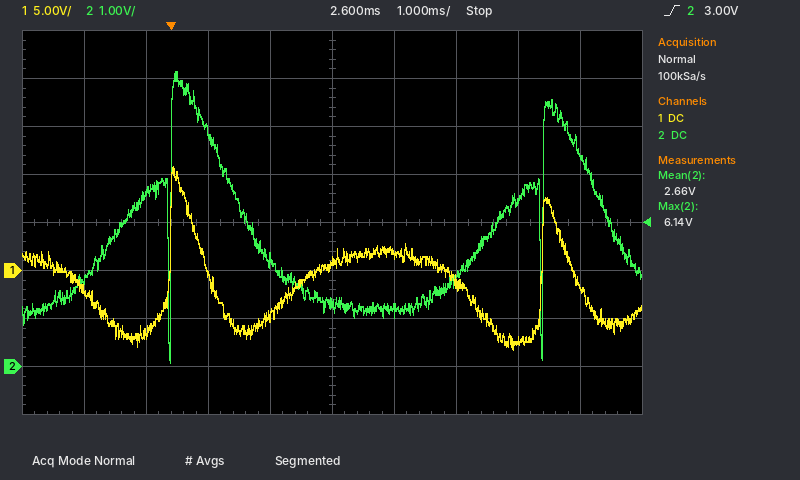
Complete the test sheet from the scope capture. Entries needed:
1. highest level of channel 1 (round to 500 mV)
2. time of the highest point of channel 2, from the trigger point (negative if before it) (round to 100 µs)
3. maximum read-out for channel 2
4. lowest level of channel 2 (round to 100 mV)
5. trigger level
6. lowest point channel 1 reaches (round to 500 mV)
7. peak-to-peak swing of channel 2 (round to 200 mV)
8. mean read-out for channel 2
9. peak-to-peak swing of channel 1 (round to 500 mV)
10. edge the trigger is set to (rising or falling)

11.0 V
+100 µs
6.14 V
100 mV
3.00 V
-8.0 V
6.0 V
2.66 V
19.0 V
rising
